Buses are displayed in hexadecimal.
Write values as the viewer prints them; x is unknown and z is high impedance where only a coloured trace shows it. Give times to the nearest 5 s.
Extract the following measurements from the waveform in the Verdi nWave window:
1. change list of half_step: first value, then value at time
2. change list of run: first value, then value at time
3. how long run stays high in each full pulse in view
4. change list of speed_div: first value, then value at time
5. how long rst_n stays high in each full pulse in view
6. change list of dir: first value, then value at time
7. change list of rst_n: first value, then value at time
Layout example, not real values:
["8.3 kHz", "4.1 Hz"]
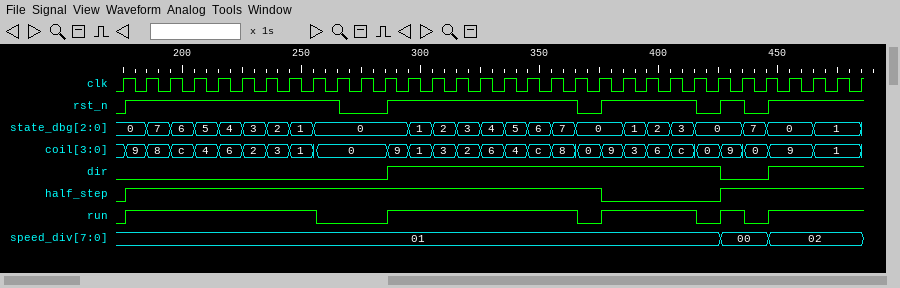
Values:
["0, 1 at 175 s, 0 at 375 s, 1 at 425 s", "0, 1 at 175 s, 0 at 255 s, 1 at 285 s, 0 at 365 s, 1 at 375 s, 0 at 415 s, 1 at 425 s, 0 at 435 s, 1 at 445 s", "80 s, 80 s, 40 s, 10 s", "01, 00 at 425 s, 02 at 445 s", "90 s, 80 s, 40 s, 10 s", "0, 1 at 285 s, 0 at 425 s, 1 at 445 s", "0, 1 at 175 s, 0 at 265 s, 1 at 285 s, 0 at 365 s, 1 at 375 s, 0 at 415 s, 1 at 425 s, 0 at 435 s, 1 at 445 s"]
